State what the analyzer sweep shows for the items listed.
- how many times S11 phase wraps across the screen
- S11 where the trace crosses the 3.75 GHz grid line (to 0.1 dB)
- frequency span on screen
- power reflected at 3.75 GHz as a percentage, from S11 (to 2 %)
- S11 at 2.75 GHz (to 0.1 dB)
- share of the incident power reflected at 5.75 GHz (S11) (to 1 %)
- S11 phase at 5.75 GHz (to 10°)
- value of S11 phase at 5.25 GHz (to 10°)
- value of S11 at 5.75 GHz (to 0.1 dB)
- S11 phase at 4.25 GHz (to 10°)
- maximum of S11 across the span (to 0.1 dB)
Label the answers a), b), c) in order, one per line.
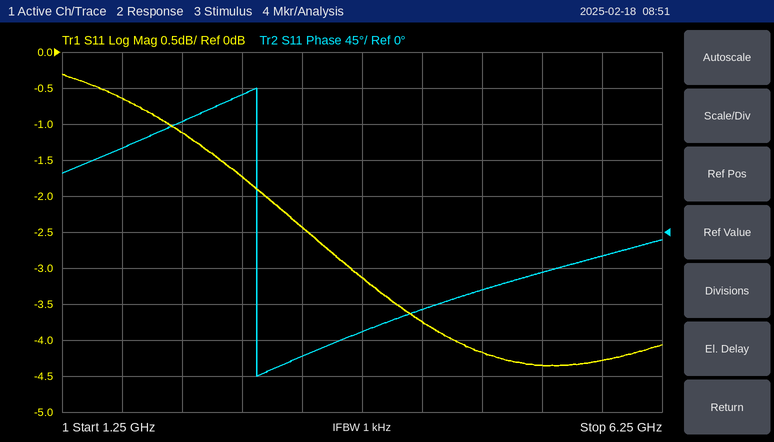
a) 1
b) -3.1 dB
c) 5 GHz
d) 48 %
e) -1.7 dB
f) 37 %
g) -30°
h) -50°
i) -4.3 dB
j) -100°
k) -0.3 dB
